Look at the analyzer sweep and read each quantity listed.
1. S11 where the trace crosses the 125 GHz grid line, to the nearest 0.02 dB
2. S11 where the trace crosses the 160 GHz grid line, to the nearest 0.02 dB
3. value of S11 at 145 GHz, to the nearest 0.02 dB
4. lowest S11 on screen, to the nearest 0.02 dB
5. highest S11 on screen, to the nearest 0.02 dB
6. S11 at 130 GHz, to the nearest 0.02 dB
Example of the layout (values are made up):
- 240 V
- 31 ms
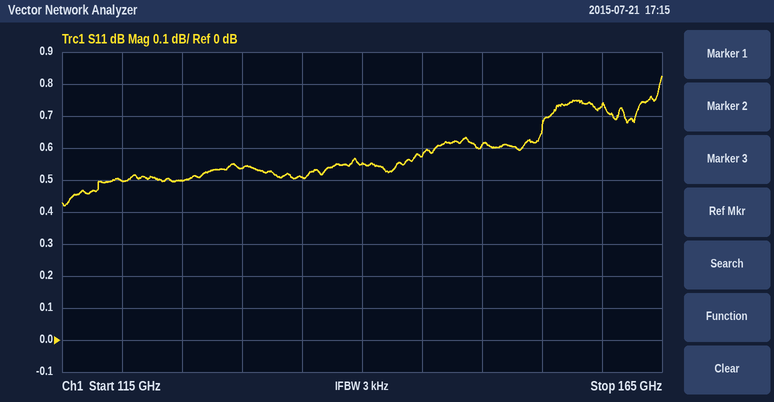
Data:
- 0.50 dB
- 0.74 dB
- 0.58 dB
- 0.42 dB
- 0.82 dB
- 0.54 dB
